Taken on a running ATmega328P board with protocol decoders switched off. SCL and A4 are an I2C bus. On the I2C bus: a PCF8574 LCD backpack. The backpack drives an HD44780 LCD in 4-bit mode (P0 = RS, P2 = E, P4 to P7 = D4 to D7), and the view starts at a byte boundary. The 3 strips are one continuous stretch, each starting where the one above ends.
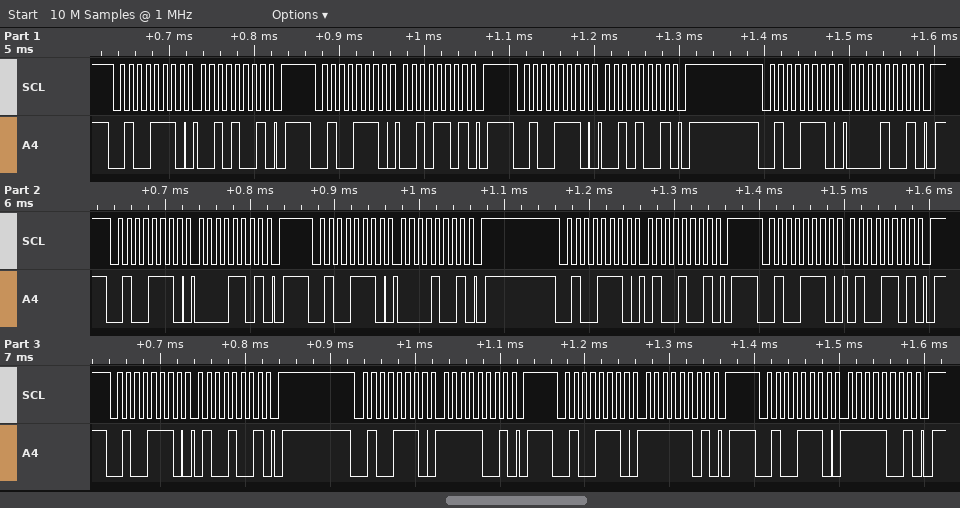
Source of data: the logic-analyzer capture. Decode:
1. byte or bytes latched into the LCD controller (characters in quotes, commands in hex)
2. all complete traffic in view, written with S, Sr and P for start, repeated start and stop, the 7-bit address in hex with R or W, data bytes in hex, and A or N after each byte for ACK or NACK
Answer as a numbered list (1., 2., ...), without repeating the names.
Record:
1. ' ' 'O'
2. S 27W A 29 A P S 27W A 2D A P S 27W A 29 A P S 27W A 09 A P S 27W A 0D A P S 27W A 09 A P S 27W A 49 A P S 27W A 4D A P S 27W A 49 A P S 27W A F9 A P S 27W A FD A P S 27W A F9 A P
